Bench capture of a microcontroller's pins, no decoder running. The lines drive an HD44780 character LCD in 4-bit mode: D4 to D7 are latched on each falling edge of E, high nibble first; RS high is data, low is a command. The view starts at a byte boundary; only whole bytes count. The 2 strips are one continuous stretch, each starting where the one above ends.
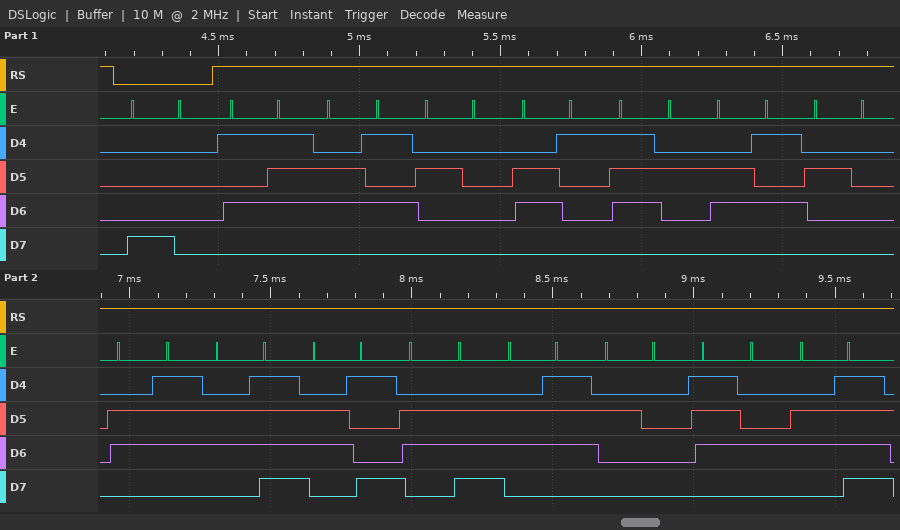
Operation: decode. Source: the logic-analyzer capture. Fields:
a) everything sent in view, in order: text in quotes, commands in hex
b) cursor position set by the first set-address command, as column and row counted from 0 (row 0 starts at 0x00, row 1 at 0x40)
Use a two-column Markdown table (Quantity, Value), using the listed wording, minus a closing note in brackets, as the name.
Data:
| Quantity | Value |
|---|---|
| everything sent in view, in order: text in quotes, commands in hex | 0x80 "We are going to" |
| cursor position set by the first set-address command, as column and row counted from 0 | column 0, row 0 |
